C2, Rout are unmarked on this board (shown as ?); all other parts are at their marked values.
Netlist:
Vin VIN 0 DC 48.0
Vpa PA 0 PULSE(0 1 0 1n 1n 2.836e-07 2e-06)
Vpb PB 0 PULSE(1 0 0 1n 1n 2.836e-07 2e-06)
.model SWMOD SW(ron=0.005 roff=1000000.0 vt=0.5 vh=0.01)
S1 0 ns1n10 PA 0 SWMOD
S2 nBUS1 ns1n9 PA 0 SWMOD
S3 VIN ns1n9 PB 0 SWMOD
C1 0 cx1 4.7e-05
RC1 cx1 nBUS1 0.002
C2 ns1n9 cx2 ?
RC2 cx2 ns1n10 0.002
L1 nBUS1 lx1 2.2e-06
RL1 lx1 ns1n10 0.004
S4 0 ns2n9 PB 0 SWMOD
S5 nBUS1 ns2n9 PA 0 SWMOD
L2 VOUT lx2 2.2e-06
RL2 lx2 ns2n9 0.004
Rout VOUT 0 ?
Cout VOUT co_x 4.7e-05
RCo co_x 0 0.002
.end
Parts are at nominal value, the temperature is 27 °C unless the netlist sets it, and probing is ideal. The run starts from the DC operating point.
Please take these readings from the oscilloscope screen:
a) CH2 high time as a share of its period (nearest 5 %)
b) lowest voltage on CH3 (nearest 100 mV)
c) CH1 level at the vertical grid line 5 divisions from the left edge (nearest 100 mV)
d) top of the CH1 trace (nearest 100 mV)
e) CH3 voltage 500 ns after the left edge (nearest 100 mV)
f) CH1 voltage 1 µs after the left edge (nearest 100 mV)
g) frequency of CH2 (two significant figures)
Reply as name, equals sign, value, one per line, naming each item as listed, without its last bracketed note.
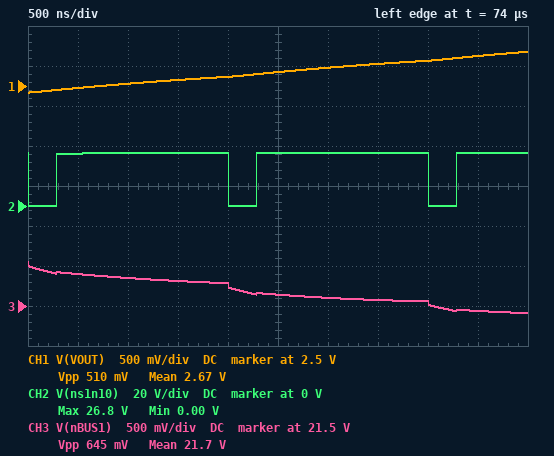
CH2 high time as a share of its period = 85 %
lowest voltage on CH3 = 21.4 V
CH1 level at the vertical grid line 5 divisions from the left edge = 2.7 V
top of the CH1 trace = 2.9 V
CH3 voltage 500 ns after the left edge = 21.9 V
CH1 voltage 1 µs after the left edge = 2.5 V
frequency of CH2 = 500 kHz
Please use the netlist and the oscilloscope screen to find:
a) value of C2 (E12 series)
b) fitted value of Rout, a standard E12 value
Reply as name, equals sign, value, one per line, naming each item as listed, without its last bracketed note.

value of C2 = 18 µF
fitted value of Rout, a standard E12 value = 0.82 Ω
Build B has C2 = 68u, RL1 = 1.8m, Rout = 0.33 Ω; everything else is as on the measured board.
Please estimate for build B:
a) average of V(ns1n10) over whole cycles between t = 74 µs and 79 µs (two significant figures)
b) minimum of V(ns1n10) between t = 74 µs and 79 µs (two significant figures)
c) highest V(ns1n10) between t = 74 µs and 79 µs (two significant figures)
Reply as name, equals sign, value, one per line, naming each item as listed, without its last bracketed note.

average of V(ns1n10) over whole cycles between t = 74 µs and 79 µs = 24 V
minimum of V(ns1n10) between t = 74 µs and 79 µs = -130 mV
highest V(ns1n10) between t = 74 µs and 79 µs = 28 V
